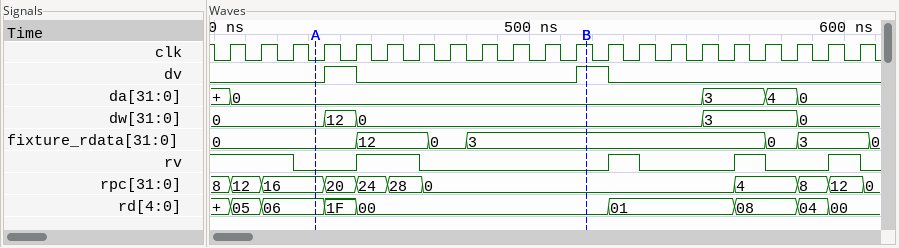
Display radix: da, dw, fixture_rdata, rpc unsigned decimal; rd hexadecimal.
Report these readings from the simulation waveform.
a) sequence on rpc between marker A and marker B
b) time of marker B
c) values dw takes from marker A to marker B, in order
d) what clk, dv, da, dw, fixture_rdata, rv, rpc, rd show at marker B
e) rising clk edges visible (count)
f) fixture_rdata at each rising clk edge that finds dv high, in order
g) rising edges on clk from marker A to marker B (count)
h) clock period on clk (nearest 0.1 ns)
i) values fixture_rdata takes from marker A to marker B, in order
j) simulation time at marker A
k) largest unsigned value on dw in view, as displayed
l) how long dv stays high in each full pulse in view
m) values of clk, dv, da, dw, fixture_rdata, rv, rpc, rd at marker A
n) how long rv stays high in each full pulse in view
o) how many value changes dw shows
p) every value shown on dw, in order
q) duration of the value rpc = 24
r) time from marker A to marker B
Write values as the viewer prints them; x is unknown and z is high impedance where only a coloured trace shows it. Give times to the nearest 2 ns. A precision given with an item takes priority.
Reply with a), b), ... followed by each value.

a) 16, 20, 24, 28, 0
b) 518 ns
c) 0, 12, 0
d) clk=1, dv=1, da=0, dw=0, fixture_rdata=3, rv=0, rpc=0, rd=00
e) 21
f) 0, 3
g) 9
h) 10 ns
i) 0, 12, 0, 3
j) 432 ns
k) 12
l) 10 ns, 10 ns
m) clk=0, dv=0, da=0, dw=0, fixture_rdata=0, rv=0, rpc=16, rd=06
n) 20 ns, 10 ns, 10 ns, 10 ns
o) 4
p) 0, 12, 0, 3, 0
q) 10 ns
r) 86 ns
